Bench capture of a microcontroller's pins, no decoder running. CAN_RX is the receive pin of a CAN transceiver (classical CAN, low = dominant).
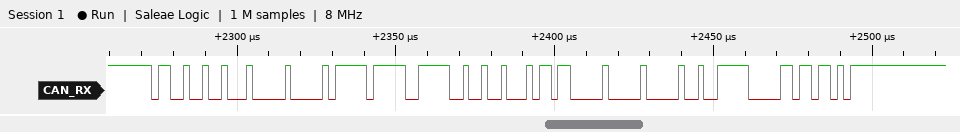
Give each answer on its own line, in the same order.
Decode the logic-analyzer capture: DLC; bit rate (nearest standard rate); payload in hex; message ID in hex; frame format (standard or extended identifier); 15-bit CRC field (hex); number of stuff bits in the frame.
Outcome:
8
500 kbit/s
00 FF DF 49 16 C0 00 13
0x649
standard
0x70B6
10
